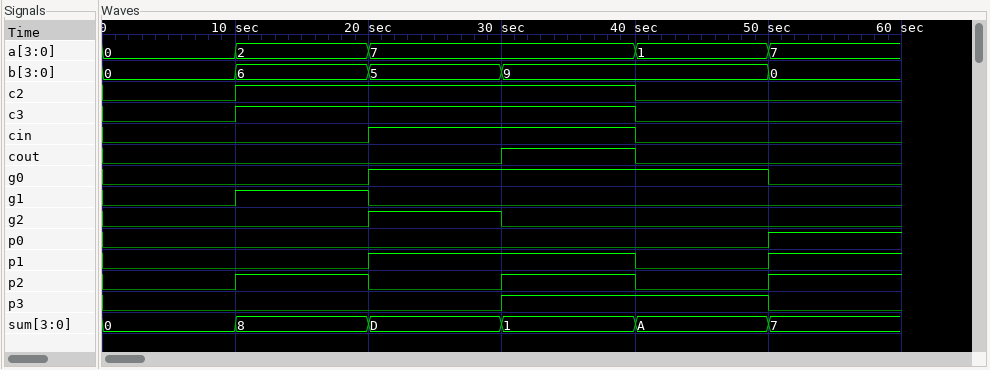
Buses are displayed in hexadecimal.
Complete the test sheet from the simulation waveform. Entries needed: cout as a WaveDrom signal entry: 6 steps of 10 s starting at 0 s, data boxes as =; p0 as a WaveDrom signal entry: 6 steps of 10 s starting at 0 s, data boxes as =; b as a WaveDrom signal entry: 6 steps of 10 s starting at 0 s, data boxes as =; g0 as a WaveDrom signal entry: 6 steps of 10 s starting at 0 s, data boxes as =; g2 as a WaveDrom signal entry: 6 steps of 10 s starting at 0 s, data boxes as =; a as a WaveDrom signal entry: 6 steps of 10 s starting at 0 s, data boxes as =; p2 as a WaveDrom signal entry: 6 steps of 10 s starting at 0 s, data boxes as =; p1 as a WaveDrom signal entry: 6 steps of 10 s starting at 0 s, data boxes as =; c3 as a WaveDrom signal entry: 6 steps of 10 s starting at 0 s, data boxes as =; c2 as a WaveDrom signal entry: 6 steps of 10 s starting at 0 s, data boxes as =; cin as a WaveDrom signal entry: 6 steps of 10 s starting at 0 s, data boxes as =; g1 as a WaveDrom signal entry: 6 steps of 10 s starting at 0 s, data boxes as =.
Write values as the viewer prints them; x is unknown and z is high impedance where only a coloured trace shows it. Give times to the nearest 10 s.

{name: 'cout', wave: '0..10.'}
{name: 'p0', wave: '0....1'}
{name: 'b', wave: '====.=', data: '0 6 5 9 0'}
{name: 'g0', wave: '0.1..0'}
{name: 'g2', wave: '0.10..'}
{name: 'a', wave: '===.==', data: '0 2 7 1 7'}
{name: 'p2', wave: '010101'}
{name: 'p1', wave: '0.1.01'}
{name: 'c3', wave: '01..0.'}
{name: 'c2', wave: '01..0.'}
{name: 'cin', wave: '0.1.0.'}
{name: 'g1', wave: '010...'}
